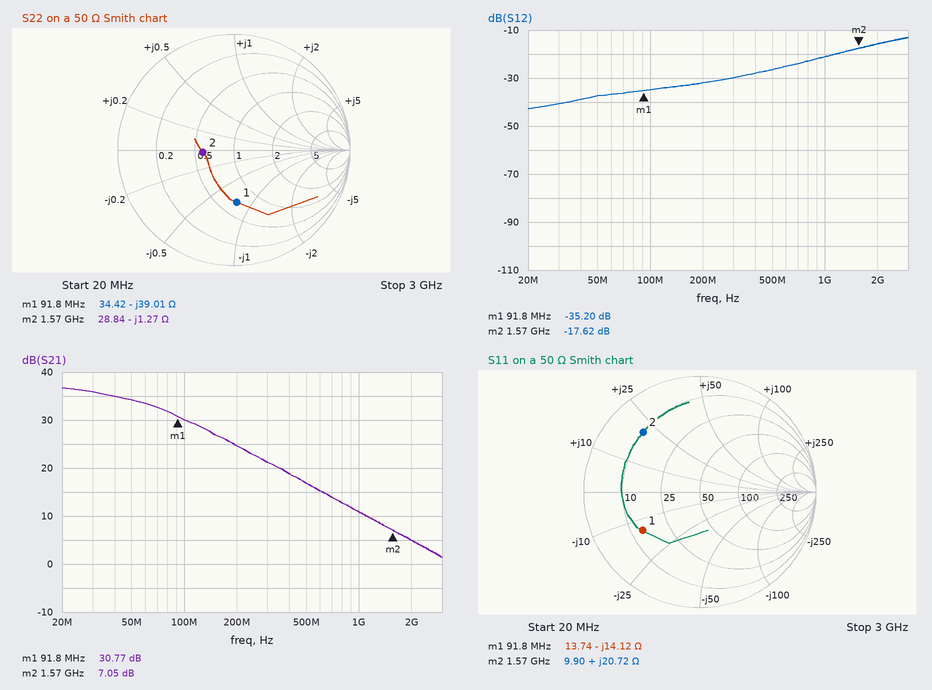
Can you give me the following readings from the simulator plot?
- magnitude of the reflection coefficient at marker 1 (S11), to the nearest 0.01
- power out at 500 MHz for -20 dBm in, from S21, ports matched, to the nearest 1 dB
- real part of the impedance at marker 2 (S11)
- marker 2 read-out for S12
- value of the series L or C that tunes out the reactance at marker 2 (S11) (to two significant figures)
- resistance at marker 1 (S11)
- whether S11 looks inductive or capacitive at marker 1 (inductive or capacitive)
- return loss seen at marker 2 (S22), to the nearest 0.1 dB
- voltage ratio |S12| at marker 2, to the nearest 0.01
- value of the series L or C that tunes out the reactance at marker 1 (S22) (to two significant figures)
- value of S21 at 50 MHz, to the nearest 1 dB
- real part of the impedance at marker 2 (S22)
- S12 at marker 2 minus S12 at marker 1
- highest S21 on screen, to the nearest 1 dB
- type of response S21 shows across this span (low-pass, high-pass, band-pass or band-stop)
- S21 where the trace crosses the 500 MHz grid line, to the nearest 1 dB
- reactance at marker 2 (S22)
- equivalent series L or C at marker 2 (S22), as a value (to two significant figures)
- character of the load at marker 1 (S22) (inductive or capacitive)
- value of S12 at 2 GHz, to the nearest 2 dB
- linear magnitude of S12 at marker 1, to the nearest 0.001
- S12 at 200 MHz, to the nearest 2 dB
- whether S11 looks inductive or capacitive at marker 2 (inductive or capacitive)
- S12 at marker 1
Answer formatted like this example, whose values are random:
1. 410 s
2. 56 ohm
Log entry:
1. 0.60
2. -3 dBm
3. 9.90 Ω
4. -17.62 dB
5. 4.9 pF
6. 13.74 Ω
7. capacitive
8. 11.4 dB
9. 0.13
10. 68 nH
11. 34 dB
12. 28.84 Ω
13. 17.58 dB
14. 37 dB
15. low-pass
16. 17 dB
17. -1.27 Ω
18. 80 pF
19. capacitive
20. -16 dB
21. 0.017
22. -32 dB
23. inductive
24. -35.20 dB
